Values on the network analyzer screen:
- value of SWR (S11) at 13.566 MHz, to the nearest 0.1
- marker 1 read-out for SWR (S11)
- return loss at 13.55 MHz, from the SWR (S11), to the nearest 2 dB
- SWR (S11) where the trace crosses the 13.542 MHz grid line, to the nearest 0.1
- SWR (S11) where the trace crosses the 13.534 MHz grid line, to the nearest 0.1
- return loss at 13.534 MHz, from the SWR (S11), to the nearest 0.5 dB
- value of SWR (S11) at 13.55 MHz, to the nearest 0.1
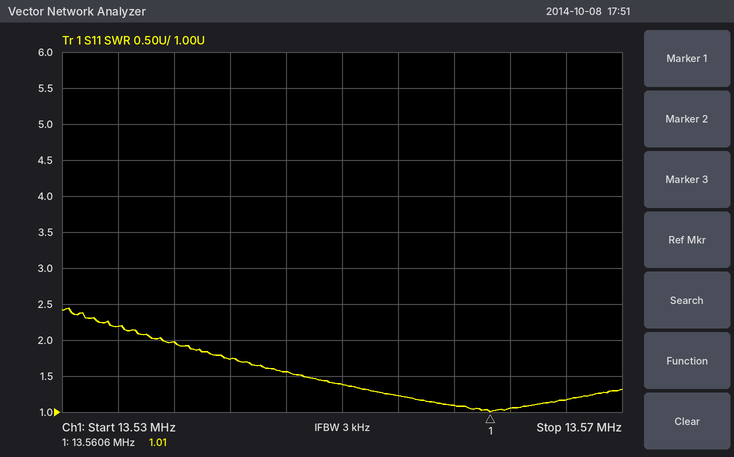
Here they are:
1.2
1.01
16 dB
1.7
2.2
8.5 dB
1.4
